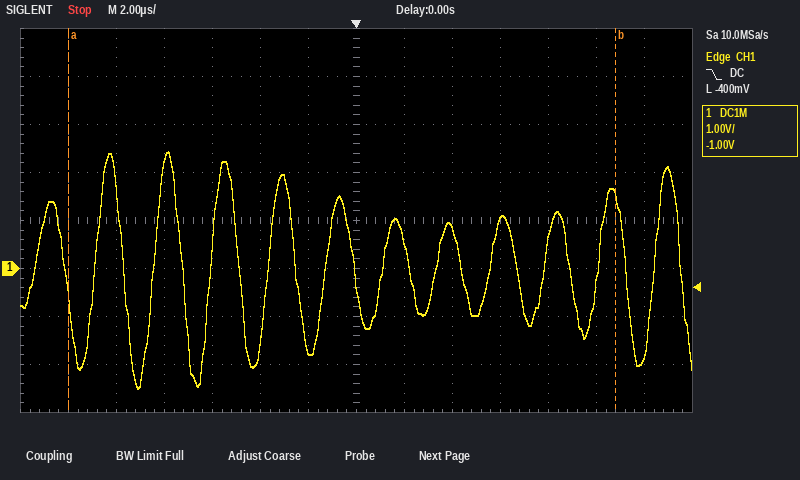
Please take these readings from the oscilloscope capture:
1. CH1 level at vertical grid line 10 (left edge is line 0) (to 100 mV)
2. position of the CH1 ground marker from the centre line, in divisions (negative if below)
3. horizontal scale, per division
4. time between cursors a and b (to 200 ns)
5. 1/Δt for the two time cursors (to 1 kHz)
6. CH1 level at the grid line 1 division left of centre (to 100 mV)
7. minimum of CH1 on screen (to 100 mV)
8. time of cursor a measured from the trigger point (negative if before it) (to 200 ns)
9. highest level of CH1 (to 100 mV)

1.0 V
-1.0 div
2 µs
22.8 µs
44 kHz
-1.7 V
-2.5 V
-12.0 µs
2.4 V
